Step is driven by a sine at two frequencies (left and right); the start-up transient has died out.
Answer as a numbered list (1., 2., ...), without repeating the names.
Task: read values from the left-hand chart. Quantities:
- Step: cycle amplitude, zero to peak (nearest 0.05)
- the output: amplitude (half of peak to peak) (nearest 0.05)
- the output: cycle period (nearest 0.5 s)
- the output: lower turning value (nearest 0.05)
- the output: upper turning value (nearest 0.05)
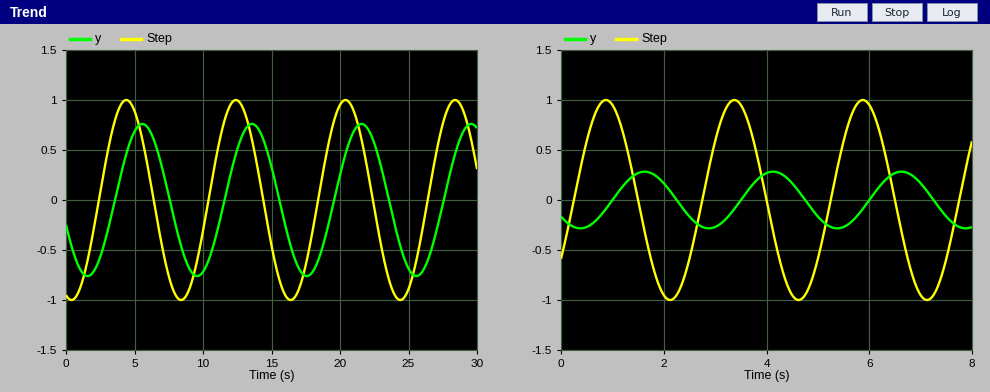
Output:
1. 1.00
2. 0.75
3. 8.0 s
4. -0.75
5. 0.75
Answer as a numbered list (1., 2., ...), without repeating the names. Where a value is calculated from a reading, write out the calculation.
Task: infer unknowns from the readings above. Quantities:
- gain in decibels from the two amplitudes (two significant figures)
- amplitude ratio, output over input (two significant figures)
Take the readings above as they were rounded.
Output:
1. 20 log10(0.75 / 1) = -2.5 dB
2. 0.75 / 1 = 0.75
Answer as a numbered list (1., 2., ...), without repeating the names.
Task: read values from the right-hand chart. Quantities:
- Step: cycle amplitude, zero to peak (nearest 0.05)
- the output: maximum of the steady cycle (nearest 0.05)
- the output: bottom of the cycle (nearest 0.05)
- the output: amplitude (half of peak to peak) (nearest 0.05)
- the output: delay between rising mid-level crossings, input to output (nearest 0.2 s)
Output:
1. 1.00
2. 0.30
3. -0.30
4. 0.30
5. 0.8 s
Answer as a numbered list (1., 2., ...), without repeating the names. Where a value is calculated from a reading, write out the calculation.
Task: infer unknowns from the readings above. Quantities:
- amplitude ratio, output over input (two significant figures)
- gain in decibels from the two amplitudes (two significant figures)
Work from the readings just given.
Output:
1. 0.3 / 1 = 0.30
2. 20 log10(0.3 / 1) = -10 dB
